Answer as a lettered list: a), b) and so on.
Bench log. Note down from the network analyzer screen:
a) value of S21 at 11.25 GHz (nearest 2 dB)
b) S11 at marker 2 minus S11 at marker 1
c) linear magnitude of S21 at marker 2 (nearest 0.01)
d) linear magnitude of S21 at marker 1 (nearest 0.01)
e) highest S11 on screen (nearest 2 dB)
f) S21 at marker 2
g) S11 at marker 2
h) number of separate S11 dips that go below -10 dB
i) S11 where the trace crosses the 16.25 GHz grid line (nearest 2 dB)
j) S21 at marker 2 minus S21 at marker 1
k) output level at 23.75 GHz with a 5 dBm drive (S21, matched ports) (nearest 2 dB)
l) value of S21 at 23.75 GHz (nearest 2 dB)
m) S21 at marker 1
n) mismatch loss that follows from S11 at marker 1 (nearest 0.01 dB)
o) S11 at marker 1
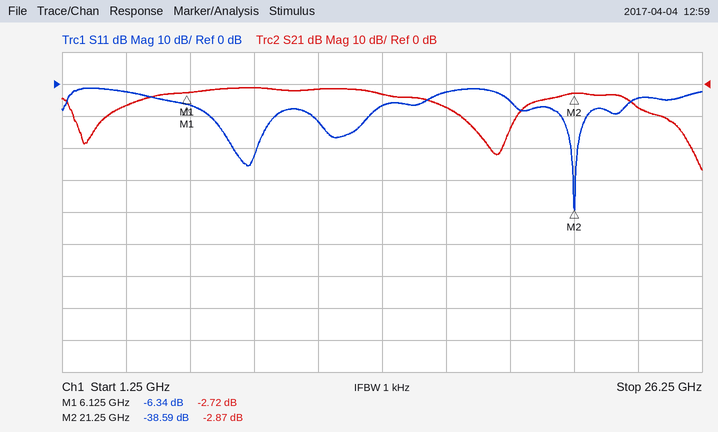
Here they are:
a) -2 dB
b) -32.25 dB
c) 0.72
d) 0.73
e) -2 dB
f) -2.87 dB
g) -38.59 dB
h) 3
i) -2 dB
j) -0.15 dB
k) -2 dBm
l) -8 dB
m) -2.72 dB
n) 1.15 dB
o) -6.34 dB
